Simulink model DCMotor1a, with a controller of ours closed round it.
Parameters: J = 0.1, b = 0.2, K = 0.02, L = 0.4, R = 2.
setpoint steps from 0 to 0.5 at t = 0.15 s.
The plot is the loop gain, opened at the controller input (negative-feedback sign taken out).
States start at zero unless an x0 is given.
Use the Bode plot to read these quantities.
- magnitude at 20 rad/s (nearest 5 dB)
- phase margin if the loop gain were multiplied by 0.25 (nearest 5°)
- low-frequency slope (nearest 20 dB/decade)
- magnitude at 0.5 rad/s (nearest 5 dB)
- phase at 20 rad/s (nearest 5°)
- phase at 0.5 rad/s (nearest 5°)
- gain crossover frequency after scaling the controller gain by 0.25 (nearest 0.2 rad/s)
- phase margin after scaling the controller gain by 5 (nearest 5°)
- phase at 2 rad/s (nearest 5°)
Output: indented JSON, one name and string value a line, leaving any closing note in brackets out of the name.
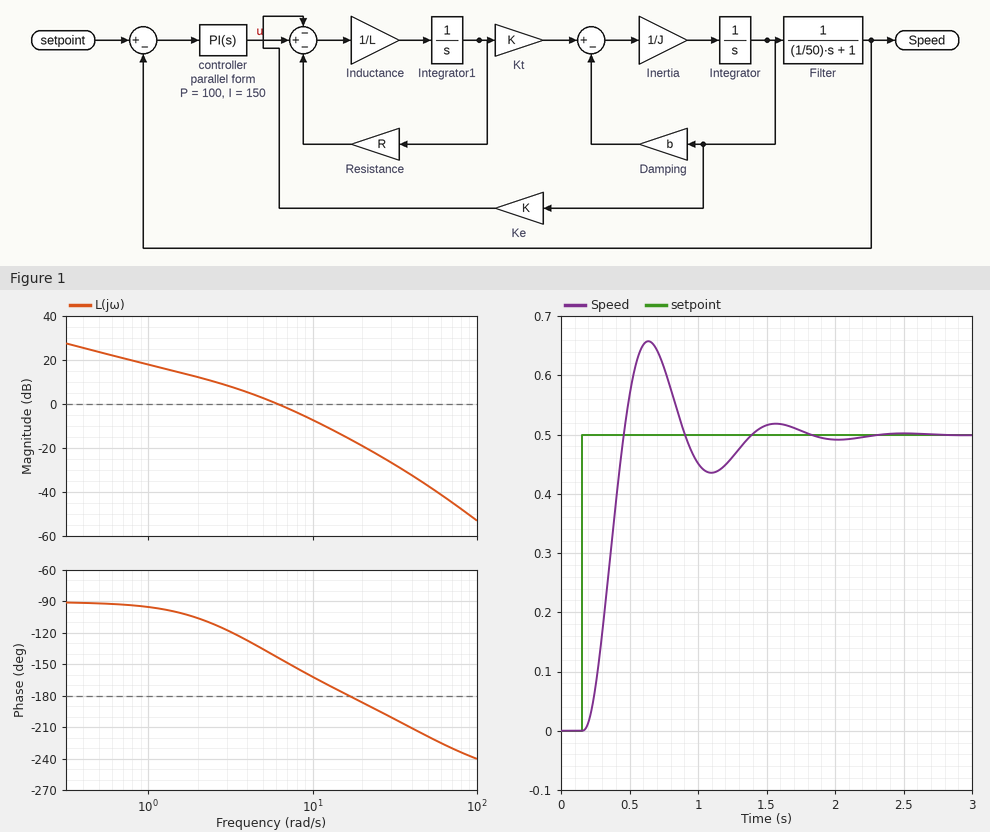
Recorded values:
{
  "magnitude at 20 rad/s": "-20 dB",
  "phase margin if the loop gain were multiplied by 0.25": "75°",
  "low-frequency slope": "-20 dB/decade",
  "magnitude at 0.5 rad/s": "25 dB",
  "phase at 20 rad/s": "-185°",
  "phase at 0.5 rad/s": "-90°",
  "gain crossover frequency after scaling the controller gain by 0.25": "2.0 rad/s",
  "phase margin after scaling the controller gain by 5": "5°",
  "phase at 2 rad/s": "-105°"
}
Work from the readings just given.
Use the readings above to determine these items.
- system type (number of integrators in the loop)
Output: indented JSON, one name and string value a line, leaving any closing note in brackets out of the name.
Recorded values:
{
  "system type": "1"
}
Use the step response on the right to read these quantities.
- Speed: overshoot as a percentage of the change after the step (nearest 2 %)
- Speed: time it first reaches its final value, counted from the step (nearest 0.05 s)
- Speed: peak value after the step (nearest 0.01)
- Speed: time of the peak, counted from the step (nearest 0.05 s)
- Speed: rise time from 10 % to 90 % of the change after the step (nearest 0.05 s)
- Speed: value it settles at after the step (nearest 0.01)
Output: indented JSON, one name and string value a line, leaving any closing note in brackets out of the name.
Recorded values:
{
  "Speed: overshoot as a percentage of the change after the step": "32 %",
  "Speed: time it first reaches its final value, counted from the step": "0.30 s",
  "Speed: peak value after the step": "0.66",
  "Speed: time of the peak, counted from the step": "0.50 s",
  "Speed: rise time from 10 % to 90 % of the change after the step": "0.20 s",
  "Speed: value it settles at after the step": "0.50"
}
